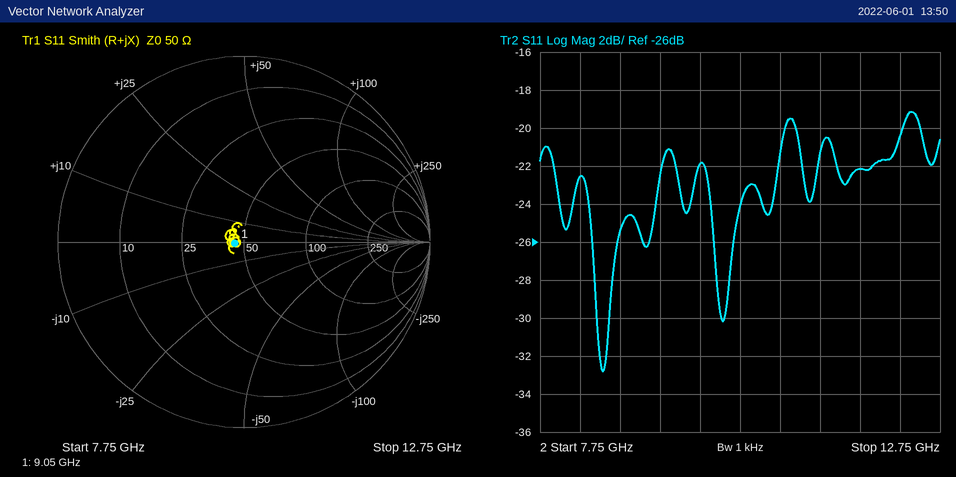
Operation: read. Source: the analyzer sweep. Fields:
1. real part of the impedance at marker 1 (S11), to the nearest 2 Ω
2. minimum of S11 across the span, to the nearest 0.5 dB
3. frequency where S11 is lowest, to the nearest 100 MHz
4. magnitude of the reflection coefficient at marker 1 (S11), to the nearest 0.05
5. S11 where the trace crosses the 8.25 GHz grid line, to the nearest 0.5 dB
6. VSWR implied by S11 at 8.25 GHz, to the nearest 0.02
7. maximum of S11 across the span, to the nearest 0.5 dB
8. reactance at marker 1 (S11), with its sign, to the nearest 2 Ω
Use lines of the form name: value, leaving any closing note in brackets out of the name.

real part of the impedance at marker 1 (S11), to the nearest 2 Ω: 46 Ω
minimum of S11 across the span, to the nearest 0.5 dB: -33.0 dB
frequency where S11 is lowest, to the nearest 100 MHz: 8.5 GHz
magnitude of the reflection coefficient at marker 1 (S11), to the nearest 0.05: 0.05
S11 where the trace crosses the 8.25 GHz grid line, to the nearest 0.5 dB: -22.5 dB
VSWR implied by S11 at 8.25 GHz, to the nearest 0.02: 1.16
maximum of S11 across the span, to the nearest 0.5 dB: -19.0 dB
reactance at marker 1 (S11), with its sign, to the nearest 2 Ω: 0 Ω
